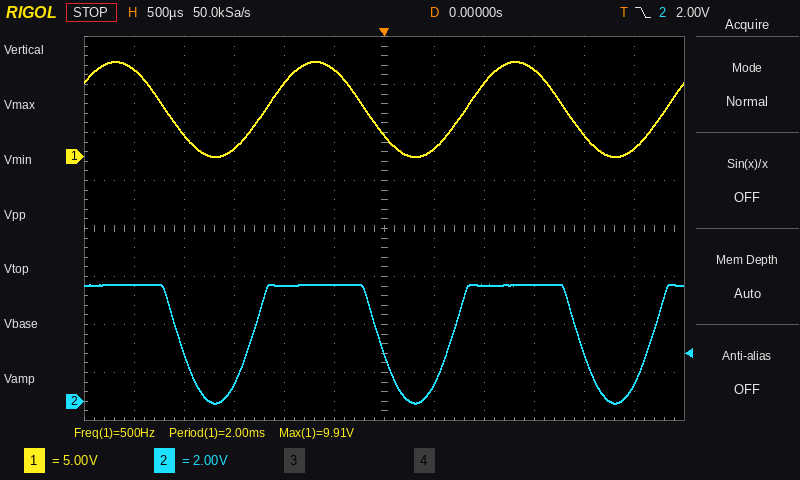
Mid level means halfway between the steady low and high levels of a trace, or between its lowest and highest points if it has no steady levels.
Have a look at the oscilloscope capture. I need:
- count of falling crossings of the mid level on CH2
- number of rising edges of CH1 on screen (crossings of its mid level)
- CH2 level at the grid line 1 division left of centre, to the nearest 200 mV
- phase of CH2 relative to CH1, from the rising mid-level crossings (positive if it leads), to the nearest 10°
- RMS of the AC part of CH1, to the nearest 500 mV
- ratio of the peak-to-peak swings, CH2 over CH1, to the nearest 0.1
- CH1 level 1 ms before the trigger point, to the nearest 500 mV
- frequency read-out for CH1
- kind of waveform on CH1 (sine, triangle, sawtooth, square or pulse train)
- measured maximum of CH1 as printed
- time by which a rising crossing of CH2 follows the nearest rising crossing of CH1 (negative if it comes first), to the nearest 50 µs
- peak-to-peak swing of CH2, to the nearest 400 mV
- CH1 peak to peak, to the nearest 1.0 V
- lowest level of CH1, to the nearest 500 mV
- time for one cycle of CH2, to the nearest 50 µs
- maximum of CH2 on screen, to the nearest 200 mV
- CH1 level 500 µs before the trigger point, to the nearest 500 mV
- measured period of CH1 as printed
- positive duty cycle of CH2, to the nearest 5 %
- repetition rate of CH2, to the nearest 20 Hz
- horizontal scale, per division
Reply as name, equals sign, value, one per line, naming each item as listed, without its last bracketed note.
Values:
count of falling crossings of the mid level on CH2 = 3
number of rising edges of CH1 on screen = 3
CH2 level at the grid line 1 division left of centre, to the nearest 200 mV = 4.8 V
phase of CH2 relative to CH1, from the rising mid-level crossings (positive if it leads), to the nearest 10° = +30°
RMS of the AC part of CH1, to the nearest 500 mV = 3.5 V
ratio of the peak-to-peak swings, CH2 over CH1, to the nearest 0.1 = 0.5
CH1 level 1 ms before the trigger point, to the nearest 500 mV = 7.5 V
frequency read-out for CH1 = 500 Hz
kind of waveform on CH1 = sine
measured maximum of CH1 as printed = 9.91 V
time by which a rising crossing of CH2 follows the nearest rising crossing of CH1 (negative if it comes first), to the nearest 50 µs = -150 µs
peak-to-peak swing of CH2, to the nearest 400 mV = 4.8 V
CH1 peak to peak, to the nearest 1.0 V = 10.0 V
lowest level of CH1, to the nearest 500 mV = 0.0 V
time for one cycle of CH2, to the nearest 50 µs = 2.00 ms
maximum of CH2 on screen, to the nearest 200 mV = 4.8 V
CH1 level 500 µs before the trigger point, to the nearest 500 mV = 9.0 V
measured period of CH1 as printed = 2.00 ms
positive duty cycle of CH2, to the nearest 5 % = 65 %
repetition rate of CH2, to the nearest 20 Hz = 500 Hz
horizontal scale, per division = 500 µs
